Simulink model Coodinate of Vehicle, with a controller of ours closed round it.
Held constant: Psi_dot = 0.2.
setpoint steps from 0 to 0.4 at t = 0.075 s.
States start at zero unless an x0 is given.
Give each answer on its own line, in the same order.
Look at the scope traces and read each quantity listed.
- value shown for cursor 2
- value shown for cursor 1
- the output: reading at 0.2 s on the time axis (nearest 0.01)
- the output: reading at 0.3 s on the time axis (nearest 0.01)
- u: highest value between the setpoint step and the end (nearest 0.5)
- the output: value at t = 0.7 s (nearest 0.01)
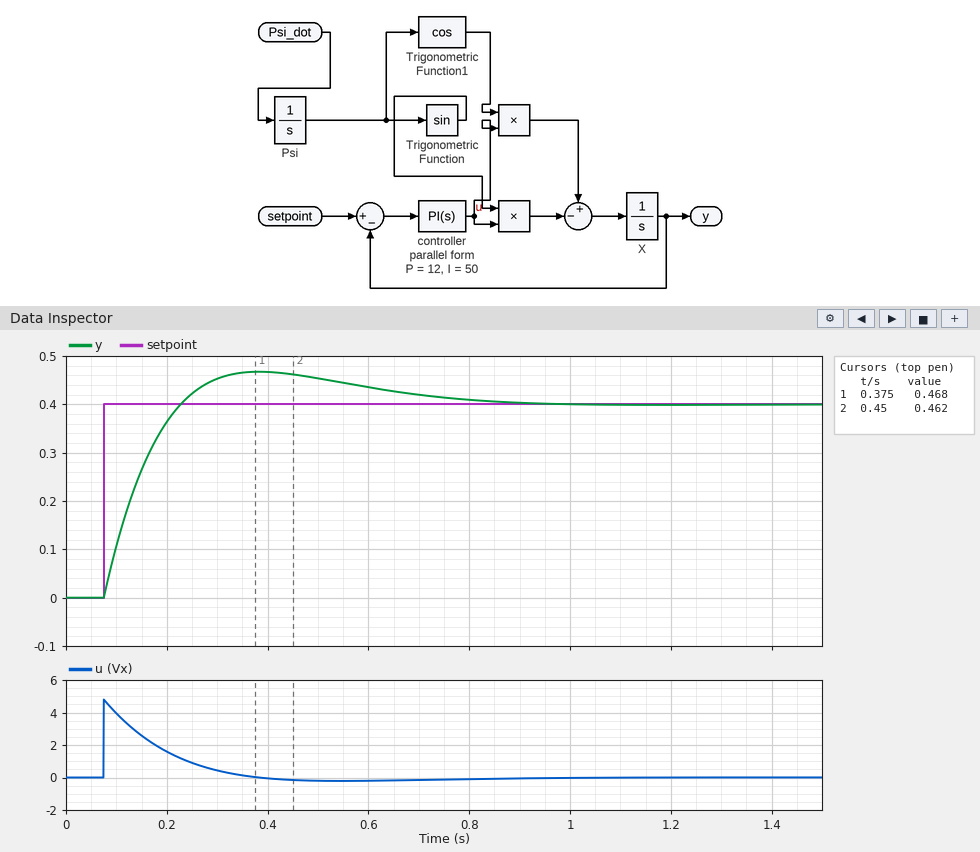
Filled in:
0.462
0.468
0.36
0.45
5.0
0.42
